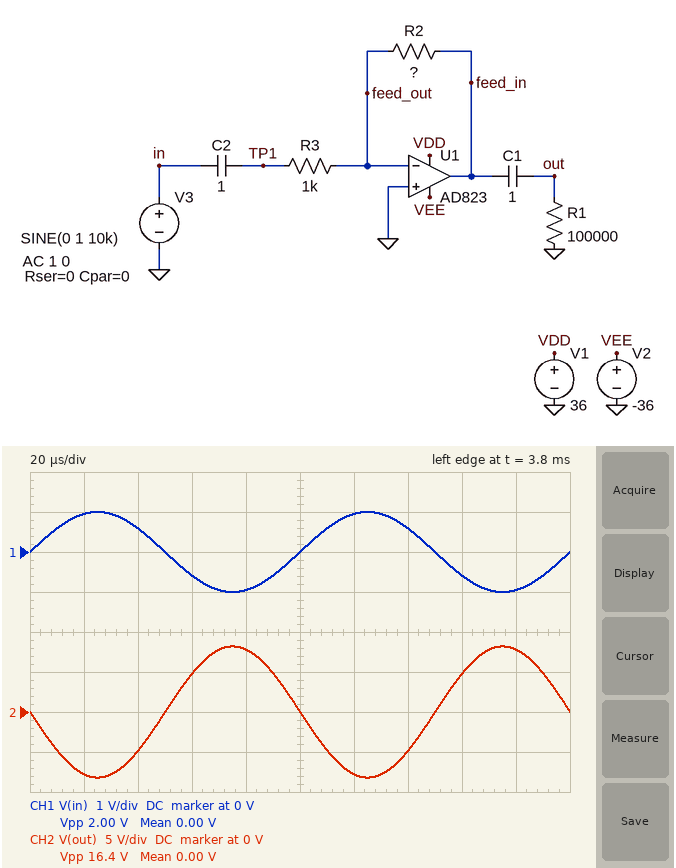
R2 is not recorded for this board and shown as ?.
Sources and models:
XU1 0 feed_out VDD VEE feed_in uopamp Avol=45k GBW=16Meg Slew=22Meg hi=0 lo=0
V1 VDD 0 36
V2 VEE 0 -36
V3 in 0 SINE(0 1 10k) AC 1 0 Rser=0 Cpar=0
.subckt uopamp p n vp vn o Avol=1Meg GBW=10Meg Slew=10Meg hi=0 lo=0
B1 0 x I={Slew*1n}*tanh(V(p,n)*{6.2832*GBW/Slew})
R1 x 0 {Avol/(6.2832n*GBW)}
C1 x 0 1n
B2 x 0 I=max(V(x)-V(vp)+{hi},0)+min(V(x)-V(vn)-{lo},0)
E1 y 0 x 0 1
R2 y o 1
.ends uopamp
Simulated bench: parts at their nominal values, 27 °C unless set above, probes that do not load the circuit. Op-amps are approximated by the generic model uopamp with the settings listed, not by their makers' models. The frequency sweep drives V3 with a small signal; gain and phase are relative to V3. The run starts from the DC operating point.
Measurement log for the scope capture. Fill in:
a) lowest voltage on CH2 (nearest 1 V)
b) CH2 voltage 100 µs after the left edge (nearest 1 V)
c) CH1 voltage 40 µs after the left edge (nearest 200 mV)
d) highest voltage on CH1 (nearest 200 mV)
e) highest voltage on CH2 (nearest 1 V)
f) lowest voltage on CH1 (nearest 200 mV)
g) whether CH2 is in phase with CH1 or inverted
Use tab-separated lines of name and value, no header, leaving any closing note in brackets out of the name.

lowest voltage on CH2	-8 V
CH2 voltage 100 µs after the left edge	0 V
CH1 voltage 40 µs after the left edge	600 mV
highest voltage on CH1	1.0 V
highest voltage on CH2	8 V
lowest voltage on CH1	-1.0 V
whether CH2 is in phase with CH1 or inverted	inverted
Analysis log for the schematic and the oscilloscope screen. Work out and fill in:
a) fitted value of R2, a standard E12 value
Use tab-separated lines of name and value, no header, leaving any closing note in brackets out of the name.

fitted value of R2, a standard E12 value	8.2 kΩ
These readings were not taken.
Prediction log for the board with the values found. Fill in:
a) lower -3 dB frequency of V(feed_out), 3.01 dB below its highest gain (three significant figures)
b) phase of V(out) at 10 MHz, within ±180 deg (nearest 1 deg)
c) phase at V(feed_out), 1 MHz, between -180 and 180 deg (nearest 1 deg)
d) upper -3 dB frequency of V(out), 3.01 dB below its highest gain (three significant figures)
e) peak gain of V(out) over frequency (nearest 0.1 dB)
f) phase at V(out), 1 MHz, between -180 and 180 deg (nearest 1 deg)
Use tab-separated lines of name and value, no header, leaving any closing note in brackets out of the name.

lower -3 dB frequency of V(feed_out), 3.01 dB below its highest gain	1.74 MHz
phase of V(out) at 10 MHz, within ±180 deg	100 deg
phase at V(feed_out), 1 MHz, between -180 and 180 deg	60 deg
upper -3 dB frequency of V(out), 3.01 dB below its highest gain	1.74 MHz
peak gain of V(out) over frequency	18.3 dB
phase at V(out), 1 MHz, between -180 and 180 deg	150 deg
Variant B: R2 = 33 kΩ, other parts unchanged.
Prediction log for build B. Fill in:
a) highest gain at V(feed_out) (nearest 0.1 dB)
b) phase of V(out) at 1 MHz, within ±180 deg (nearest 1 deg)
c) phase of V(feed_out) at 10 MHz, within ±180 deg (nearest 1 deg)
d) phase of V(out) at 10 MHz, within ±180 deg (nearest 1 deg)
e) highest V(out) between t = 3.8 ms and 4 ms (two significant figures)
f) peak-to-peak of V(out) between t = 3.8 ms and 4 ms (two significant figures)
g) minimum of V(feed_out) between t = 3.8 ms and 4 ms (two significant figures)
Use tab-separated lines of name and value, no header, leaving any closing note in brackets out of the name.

highest gain at V(feed_out)	-0.3 dB
phase of V(out) at 1 MHz, within ±180 deg	115 deg
phase of V(feed_out) at 10 MHz, within ±180 deg	3 deg
phase of V(out) at 10 MHz, within ±180 deg	93 deg
highest V(out) between t = 3.8 ms and 4 ms	33 V
peak-to-peak of V(out) between t = 3.8 ms and 4 ms	66 V
minimum of V(feed_out) between t = 3.8 ms and 4 ms	-21 mV
